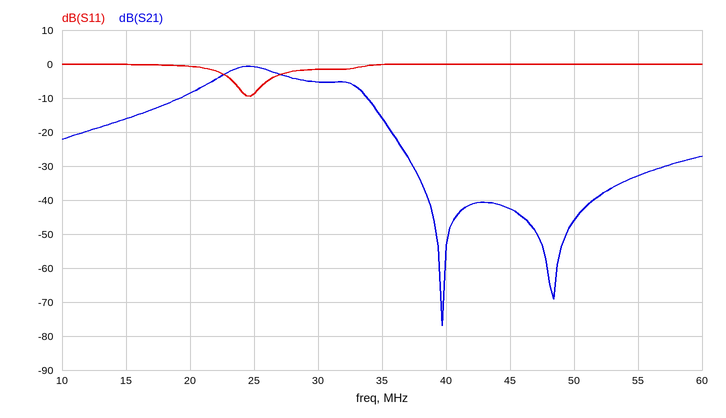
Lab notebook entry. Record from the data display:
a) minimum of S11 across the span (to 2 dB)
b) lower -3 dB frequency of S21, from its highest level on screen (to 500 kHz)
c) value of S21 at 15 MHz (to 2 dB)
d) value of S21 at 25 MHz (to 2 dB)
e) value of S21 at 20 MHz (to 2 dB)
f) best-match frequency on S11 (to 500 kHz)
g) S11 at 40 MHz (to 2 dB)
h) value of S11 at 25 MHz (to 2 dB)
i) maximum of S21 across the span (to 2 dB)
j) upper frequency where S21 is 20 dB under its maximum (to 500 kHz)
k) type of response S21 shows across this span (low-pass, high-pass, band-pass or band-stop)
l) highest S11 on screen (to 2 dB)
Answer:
-10 dB
22.5 MHz
-16 dB
0 dB
-8 dB
24.5 MHz
0 dB
-8 dB
0 dB
36.0 MHz
band-pass
0 dB
